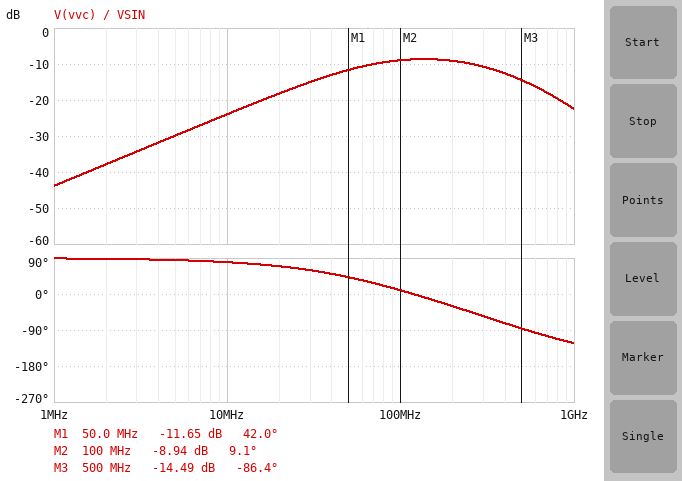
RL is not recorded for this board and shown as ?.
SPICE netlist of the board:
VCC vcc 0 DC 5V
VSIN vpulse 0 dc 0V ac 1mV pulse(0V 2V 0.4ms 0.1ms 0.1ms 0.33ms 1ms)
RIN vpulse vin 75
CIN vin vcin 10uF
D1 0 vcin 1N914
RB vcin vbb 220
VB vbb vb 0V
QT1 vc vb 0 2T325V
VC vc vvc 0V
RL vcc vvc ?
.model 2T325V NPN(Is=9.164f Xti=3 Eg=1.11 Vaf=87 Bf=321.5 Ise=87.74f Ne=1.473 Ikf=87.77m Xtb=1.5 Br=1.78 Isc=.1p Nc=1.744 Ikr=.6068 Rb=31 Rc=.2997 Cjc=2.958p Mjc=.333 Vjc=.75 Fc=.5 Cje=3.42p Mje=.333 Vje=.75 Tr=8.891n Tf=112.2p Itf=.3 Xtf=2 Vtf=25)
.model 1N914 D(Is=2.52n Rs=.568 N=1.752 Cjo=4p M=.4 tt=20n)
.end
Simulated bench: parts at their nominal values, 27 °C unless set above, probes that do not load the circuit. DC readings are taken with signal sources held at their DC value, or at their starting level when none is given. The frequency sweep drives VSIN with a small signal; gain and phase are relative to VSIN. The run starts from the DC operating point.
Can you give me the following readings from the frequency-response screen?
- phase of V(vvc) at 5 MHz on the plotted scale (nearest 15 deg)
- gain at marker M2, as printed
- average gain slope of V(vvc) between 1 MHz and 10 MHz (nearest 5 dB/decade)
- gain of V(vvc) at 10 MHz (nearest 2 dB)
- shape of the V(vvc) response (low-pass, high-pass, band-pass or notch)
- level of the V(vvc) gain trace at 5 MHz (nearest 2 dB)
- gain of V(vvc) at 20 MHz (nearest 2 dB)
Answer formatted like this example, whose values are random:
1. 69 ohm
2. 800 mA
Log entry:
1. 90 deg
2. -8.94 dB
3. 20 dB/decade
4. -24 dB
5. band-pass
6. -30 dB
7. -18 dB
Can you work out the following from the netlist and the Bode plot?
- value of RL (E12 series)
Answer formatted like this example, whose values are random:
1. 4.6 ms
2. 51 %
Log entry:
1. 680 Ω
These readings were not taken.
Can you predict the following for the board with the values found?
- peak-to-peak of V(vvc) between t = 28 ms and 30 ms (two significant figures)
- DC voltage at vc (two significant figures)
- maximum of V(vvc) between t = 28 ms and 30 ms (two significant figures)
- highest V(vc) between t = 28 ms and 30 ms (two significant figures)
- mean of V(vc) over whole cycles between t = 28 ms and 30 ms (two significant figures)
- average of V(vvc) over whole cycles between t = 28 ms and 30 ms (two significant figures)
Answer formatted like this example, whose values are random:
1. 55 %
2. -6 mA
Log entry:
1. 5.0 V
2. 5.0 V
3. 5.0 V
4. 5.0 V
5. 3.1 V
6. 3.1 V
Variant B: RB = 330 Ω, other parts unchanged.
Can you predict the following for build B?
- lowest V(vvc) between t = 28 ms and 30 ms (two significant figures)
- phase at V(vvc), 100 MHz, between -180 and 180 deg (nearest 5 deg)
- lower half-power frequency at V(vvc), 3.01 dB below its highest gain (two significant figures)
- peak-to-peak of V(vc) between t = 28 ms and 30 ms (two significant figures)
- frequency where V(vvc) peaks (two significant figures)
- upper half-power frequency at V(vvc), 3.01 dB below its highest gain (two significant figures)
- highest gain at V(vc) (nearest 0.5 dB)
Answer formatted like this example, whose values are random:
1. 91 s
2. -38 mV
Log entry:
1. 44 mV
2. 0 deg
3. 42 MHz
4. 5.0 V
5. 120 MHz
6. 320 MHz
7. -10.0 dB
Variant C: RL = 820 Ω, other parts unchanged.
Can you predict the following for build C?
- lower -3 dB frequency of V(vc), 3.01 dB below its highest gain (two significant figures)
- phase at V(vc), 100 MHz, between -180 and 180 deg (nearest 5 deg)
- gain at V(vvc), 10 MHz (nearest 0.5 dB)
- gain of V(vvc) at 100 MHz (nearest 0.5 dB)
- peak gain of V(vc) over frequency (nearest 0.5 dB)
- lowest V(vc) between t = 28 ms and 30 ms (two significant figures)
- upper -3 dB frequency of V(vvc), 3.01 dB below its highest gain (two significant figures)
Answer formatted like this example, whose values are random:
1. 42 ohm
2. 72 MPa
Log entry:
1. 46 MHz
2. 5 deg
3. -22.5 dB
4. -8.0 dB
5. -7.5 dB
6. 36 mV
7. 320 MHz
